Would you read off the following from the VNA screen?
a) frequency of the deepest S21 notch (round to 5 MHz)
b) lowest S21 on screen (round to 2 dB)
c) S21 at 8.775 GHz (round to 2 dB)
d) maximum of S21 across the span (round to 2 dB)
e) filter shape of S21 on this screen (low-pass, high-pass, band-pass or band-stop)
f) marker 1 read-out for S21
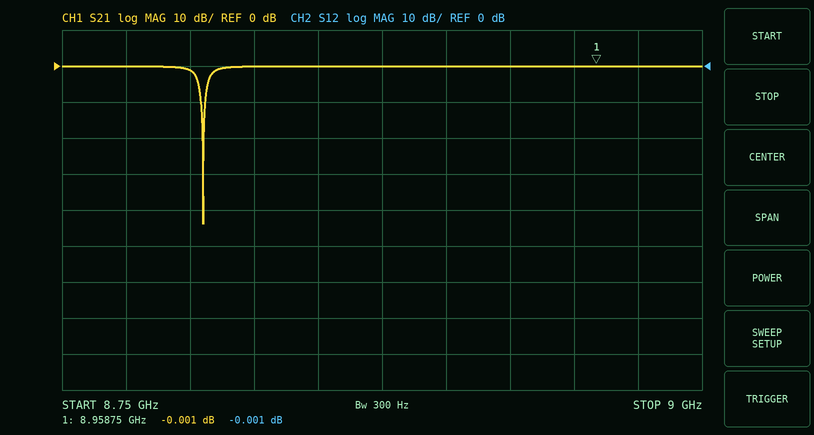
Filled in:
8.805 GHz
-44 dB
0 dB
0 dB
band-stop
-0.001 dB
